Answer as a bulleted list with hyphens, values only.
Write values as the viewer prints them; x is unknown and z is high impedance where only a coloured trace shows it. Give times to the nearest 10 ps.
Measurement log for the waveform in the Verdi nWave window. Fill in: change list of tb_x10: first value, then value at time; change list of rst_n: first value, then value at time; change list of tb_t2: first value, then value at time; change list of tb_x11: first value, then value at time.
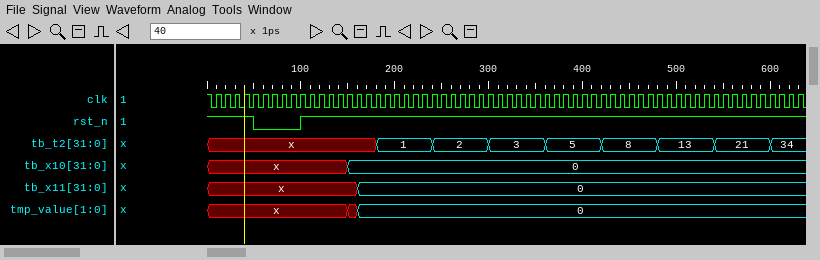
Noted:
- x, 0 at 150 ps
- 1, 0 at 50 ps, 1 at 100 ps
- x, 1 at 180 ps, 2 at 240 ps, 3 at 300 ps, 5 at 360 ps, 8 at 420 ps, 13 at 480 ps, 21 at 540 ps, 34 at 600 ps
- x, 0 at 160 ps
